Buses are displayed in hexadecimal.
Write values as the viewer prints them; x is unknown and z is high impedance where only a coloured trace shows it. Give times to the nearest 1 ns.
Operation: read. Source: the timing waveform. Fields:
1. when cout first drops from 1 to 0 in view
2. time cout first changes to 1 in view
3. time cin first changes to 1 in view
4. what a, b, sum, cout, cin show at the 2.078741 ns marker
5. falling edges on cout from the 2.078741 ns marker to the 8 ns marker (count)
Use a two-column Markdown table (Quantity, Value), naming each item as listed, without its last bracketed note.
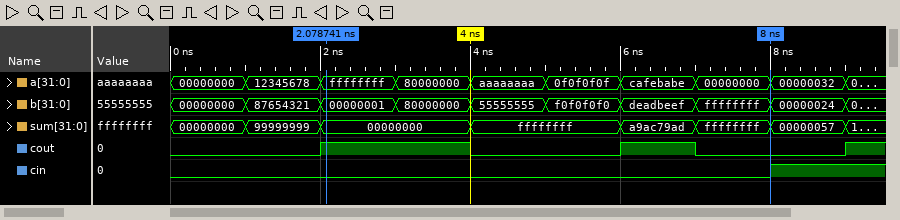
| Quantity | Value |
|---|---|
| when cout first drops from 1 to 0 in view | 4 ns |
| time cout first changes to 1 in view | 2 ns |
| time cin first changes to 1 in view | 8 ns |
| what a, b, sum, cout, cin show at the 2.078741 ns marker | a=ffffffff, b=00000001, sum=00000000, cout=1, cin=0 |
| falling edges on cout from the 2.078741 ns marker to the 8 ns marker | 2 |
